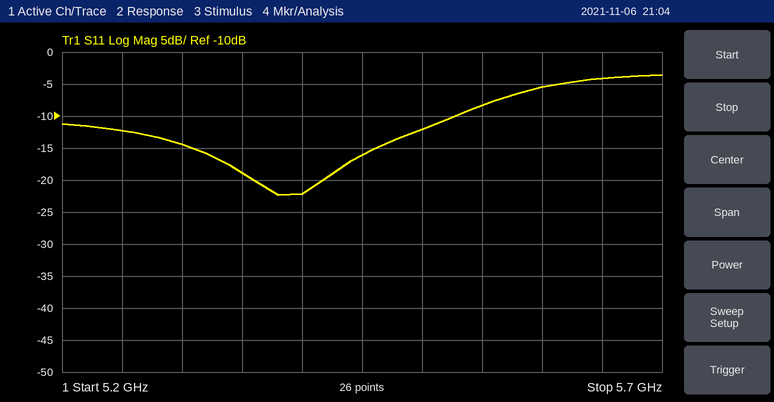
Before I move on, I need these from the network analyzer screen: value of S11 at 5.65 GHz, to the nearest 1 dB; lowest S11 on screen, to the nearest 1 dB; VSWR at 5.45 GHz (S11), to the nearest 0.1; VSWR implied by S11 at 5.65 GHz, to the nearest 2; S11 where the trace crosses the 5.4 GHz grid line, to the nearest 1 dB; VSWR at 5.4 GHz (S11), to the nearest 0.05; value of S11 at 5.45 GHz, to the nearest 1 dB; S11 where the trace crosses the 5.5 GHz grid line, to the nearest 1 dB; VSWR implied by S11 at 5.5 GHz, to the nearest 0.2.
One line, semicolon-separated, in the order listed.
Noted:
-4 dB; -22 dB; 1.4; 4; -22 dB; 1.15; -16 dB; -12 dB; 1.6
